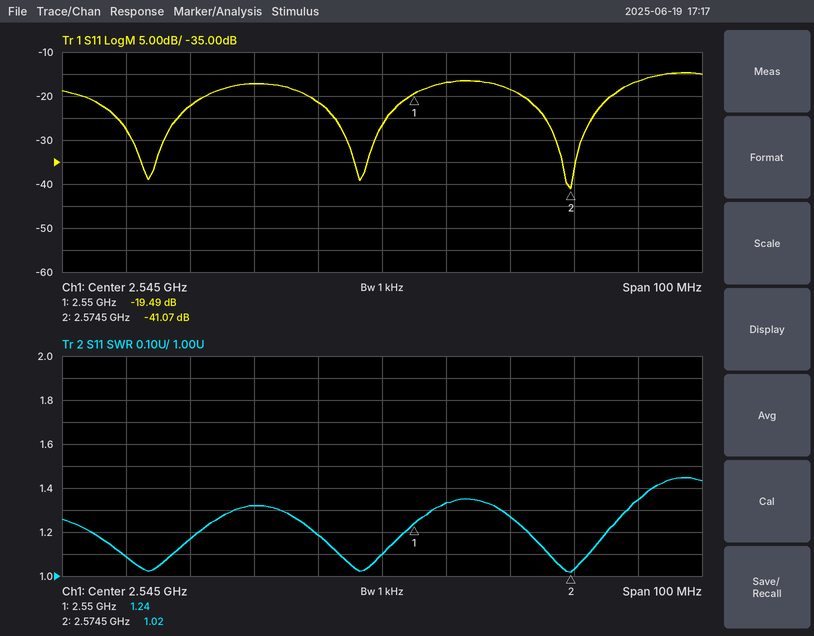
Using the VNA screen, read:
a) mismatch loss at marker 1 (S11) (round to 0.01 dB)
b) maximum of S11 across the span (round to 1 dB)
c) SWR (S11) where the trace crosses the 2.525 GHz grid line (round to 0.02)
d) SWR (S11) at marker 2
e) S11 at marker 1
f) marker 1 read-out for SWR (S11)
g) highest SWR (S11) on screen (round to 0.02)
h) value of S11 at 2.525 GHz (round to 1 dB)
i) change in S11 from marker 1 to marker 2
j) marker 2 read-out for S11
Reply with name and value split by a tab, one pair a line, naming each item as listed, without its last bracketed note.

mismatch loss at marker 1 (S11)	0.05 dB
maximum of S11 across the span	-15 dB
SWR (S11) where the trace crosses the 2.525 GHz grid line	1.32
SWR (S11) at marker 2	1.02
S11 at marker 1	-19.49 dB
marker 1 read-out for SWR	1.24
highest SWR (S11) on screen	1.44
value of S11 at 2.525 GHz	-17 dB
change in S11 from marker 1 to marker 2	-21.58 dB
marker 2 read-out for S11	-41.07 dB
